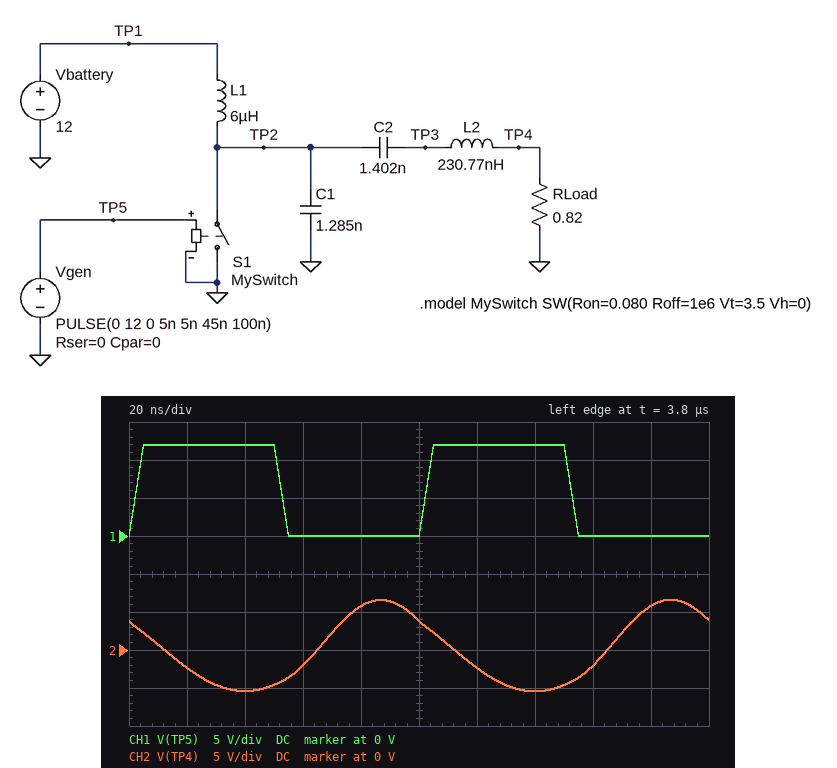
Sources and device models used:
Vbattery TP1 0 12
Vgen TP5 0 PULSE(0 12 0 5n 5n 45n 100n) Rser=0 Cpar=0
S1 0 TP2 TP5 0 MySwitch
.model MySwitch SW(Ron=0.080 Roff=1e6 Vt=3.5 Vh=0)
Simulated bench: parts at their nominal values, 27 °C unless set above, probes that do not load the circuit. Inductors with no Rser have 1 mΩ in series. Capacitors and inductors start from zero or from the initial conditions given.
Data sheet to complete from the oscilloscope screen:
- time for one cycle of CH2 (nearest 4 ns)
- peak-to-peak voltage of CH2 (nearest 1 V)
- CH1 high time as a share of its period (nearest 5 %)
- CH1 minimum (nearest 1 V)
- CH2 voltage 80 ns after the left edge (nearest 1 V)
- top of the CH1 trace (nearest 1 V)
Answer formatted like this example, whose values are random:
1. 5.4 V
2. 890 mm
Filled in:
1. 100 ns
2. 12 V
3. 50 %
4. 0 V
5. 6 V
6. 12 V
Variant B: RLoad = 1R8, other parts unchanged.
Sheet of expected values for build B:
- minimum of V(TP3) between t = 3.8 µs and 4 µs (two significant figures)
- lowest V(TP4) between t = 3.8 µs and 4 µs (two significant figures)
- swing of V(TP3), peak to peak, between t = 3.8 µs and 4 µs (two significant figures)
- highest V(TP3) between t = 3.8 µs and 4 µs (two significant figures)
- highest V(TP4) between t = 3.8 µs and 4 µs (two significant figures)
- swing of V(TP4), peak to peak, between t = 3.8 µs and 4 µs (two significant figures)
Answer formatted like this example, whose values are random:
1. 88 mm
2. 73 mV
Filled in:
1. -71 V
2. -8.9 V
3. 170 V
4. 95 V
5. 11 V
6. 20 V
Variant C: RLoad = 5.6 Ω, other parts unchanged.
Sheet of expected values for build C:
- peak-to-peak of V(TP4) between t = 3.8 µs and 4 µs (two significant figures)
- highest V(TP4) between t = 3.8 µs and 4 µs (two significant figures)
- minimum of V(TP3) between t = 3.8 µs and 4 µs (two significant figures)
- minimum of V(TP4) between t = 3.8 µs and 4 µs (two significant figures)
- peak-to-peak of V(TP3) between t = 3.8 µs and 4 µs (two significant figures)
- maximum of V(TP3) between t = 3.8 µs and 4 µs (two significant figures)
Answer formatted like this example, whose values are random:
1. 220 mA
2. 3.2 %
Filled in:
1. 29 V
2. 16 V
3. -42 V
4. -14 V
5. 88 V
6. 46 V
